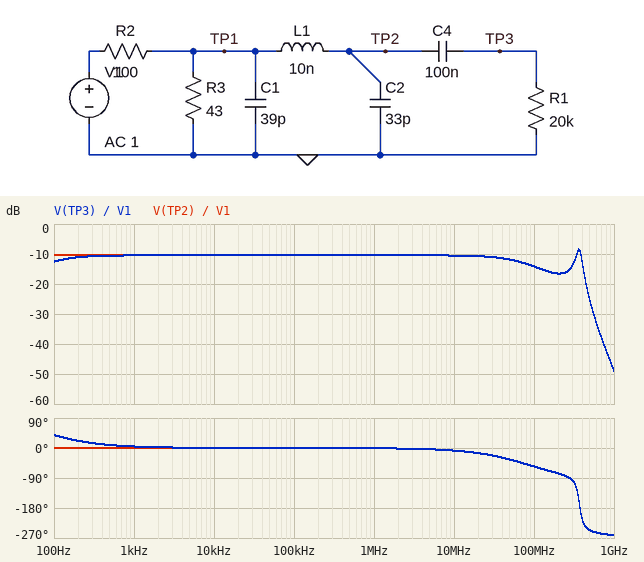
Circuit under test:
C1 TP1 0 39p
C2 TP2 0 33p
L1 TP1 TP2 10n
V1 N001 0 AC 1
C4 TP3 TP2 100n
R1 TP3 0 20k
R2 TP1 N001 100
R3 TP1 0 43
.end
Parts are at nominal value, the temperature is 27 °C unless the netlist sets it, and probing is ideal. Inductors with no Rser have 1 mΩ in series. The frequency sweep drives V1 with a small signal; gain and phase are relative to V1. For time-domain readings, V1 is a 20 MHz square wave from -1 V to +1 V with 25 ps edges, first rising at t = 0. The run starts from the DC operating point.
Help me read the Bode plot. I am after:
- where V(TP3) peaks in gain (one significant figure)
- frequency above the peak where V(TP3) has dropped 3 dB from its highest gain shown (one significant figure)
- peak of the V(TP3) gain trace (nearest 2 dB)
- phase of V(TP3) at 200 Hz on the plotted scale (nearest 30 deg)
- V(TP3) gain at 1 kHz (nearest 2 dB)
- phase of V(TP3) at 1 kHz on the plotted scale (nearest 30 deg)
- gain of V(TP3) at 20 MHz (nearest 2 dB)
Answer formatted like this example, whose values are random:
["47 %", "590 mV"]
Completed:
["400 MHz", "400 MHz", "-8 dB", "30 deg", "-10 dB", "0 deg", "-10 dB"]
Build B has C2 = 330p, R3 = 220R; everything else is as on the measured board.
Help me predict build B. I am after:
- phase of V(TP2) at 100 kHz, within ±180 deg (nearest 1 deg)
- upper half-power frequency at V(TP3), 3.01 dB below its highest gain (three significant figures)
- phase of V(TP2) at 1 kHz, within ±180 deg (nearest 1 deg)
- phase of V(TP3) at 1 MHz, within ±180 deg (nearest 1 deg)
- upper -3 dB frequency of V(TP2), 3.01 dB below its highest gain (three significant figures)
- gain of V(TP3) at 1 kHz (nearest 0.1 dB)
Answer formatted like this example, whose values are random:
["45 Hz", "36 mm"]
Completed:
["-1 deg", "6.33 MHz", "0 deg", "-9 deg", "6.29 MHz", "-3.3 dB"]
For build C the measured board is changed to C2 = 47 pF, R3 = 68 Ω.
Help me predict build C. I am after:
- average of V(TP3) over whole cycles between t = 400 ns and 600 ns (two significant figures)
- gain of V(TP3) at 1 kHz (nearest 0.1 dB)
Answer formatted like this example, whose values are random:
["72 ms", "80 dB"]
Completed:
["400 mV", "-7.9 dB"]
